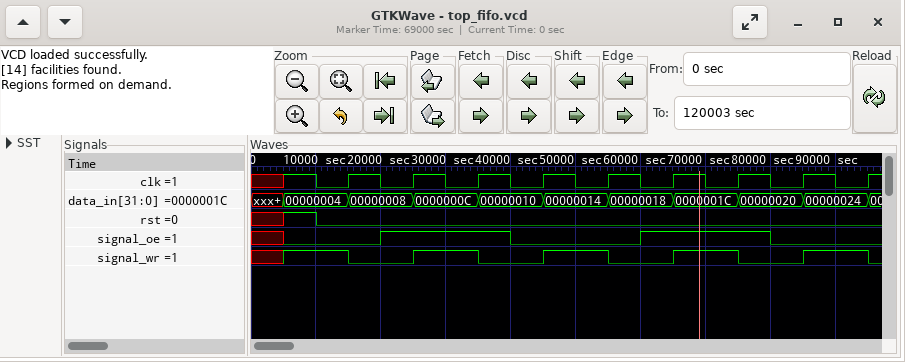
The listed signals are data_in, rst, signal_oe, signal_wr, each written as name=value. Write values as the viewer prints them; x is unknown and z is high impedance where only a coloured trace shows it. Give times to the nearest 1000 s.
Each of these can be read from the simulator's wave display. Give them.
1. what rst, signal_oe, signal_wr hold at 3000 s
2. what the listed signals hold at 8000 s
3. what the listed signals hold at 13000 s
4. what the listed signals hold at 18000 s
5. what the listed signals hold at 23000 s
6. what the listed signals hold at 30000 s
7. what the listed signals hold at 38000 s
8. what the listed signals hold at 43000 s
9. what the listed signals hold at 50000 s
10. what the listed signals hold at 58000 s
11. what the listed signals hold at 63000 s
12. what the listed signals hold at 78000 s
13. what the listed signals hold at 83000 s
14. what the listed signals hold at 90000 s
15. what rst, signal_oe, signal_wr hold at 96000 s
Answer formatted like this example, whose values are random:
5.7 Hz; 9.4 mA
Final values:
rst=x, signal_oe=x, signal_wr=x; data_in=00000004, rst=1, signal_oe=0, signal_wr=1; data_in=00000004, rst=0, signal_oe=0, signal_wr=1; data_in=00000008, rst=0, signal_oe=0, signal_wr=0; data_in=00000008, rst=0, signal_oe=1, signal_wr=0; data_in=0000000C, rst=0, signal_oe=1, signal_wr=1; data_in=00000010, rst=0, signal_oe=1, signal_wr=0; data_in=00000010, rst=0, signal_oe=0, signal_wr=0; data_in=00000014, rst=0, signal_oe=0, signal_wr=1; data_in=00000018, rst=0, signal_oe=0, signal_wr=0; data_in=00000018, rst=0, signal_oe=1, signal_wr=0; data_in=00000020, rst=0, signal_oe=1, signal_wr=0; data_in=00000020, rst=0, signal_oe=0, signal_wr=0; data_in=00000024, rst=0, signal_oe=0, signal_wr=1; rst=0, signal_oe=0, signal_wr=0
